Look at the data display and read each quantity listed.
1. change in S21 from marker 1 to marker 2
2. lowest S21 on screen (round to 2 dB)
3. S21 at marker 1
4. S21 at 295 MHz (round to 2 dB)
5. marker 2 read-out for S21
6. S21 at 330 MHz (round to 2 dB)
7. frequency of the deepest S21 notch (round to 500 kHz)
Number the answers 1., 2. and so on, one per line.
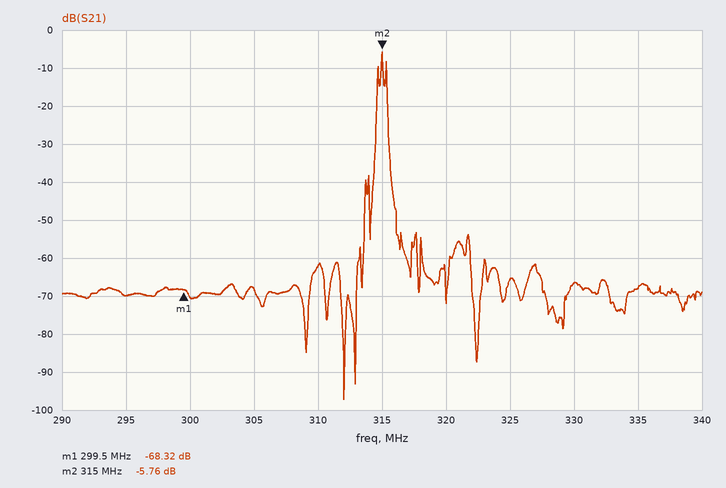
1. 62.56 dB
2. -98 dB
3. -68.32 dB
4. -70 dB
5. -5.76 dB
6. -66 dB
7. 312.0 MHz
